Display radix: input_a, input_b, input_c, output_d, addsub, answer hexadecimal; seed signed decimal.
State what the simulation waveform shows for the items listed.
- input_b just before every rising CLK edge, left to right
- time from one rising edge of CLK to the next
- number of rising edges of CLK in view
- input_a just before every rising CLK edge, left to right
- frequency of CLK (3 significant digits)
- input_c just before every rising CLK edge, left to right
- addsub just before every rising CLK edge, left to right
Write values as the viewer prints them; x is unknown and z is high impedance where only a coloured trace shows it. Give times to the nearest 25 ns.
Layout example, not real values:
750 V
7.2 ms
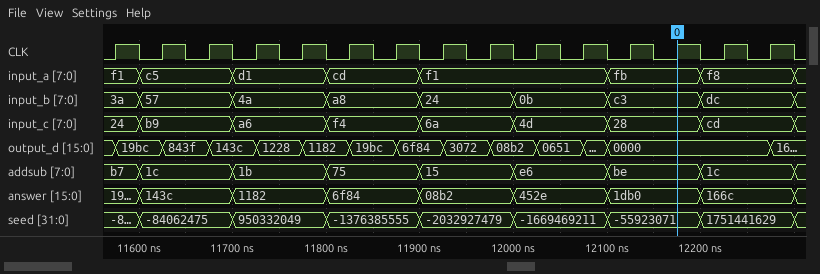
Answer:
3a, 57, 57, 4a, 4a, a8, a8, 24, 24, 0b, 0b, c3, c3, dc, dc
50 ns
15
f1, c5, c5, d1, d1, cd, cd, f1, f1, f1, f1, fb, fb, f8, f8
20.0 MHz
24, b9, b9, a6, a6, f4, f4, 6a, 6a, 4d, 4d, 28, 28, cd, cd
b7, 1c, 1c, 1b, 1b, 75, 75, 15, 15, e6, e6, be, be, 1c, 1c
